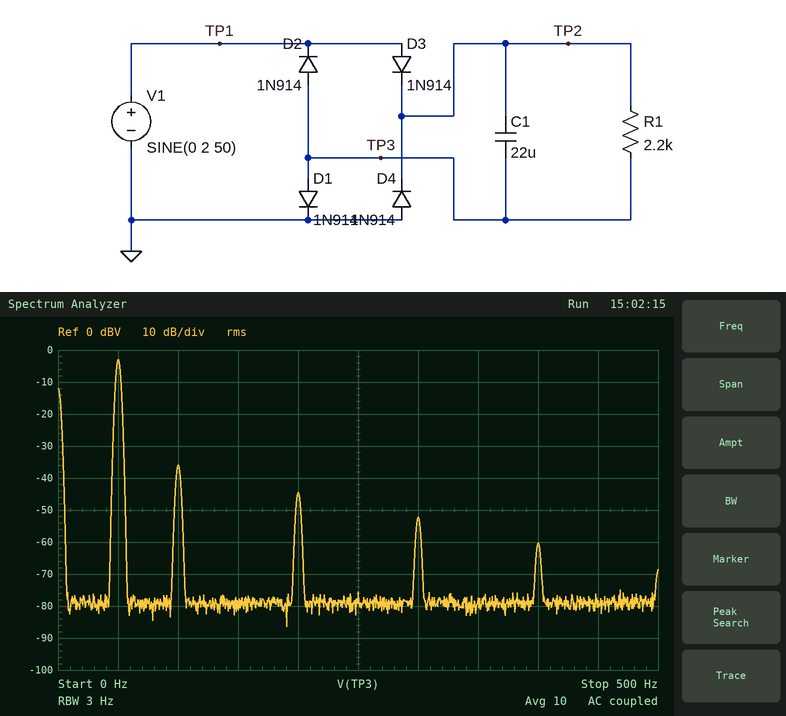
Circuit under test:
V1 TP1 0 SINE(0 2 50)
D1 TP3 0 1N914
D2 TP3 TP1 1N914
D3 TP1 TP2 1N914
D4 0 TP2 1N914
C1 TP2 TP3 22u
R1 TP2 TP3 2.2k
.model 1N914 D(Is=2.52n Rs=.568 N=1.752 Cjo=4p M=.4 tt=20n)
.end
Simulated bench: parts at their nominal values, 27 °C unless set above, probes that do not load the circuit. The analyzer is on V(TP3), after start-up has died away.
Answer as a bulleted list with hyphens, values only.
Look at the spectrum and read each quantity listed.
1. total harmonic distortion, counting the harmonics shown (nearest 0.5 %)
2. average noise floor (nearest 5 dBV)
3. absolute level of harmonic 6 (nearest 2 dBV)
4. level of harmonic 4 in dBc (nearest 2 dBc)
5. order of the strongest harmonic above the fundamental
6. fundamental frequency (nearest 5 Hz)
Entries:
- 2.5 %
- -80 dBV
- -52 dBV
- -42 dBc
- 2
- 50 Hz
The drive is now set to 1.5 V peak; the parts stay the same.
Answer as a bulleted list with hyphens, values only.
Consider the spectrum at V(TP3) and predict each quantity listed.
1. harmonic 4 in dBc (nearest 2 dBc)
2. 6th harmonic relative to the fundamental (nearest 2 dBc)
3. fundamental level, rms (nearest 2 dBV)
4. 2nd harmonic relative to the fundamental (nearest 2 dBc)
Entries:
- -46 dBc
- -56 dBc
- -6 dBV
- -38 dBc
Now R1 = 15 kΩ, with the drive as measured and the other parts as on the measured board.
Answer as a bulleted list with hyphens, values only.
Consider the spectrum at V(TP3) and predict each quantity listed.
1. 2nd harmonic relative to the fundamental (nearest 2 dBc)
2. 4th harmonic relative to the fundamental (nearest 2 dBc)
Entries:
- -48 dBc
- -56 dBc
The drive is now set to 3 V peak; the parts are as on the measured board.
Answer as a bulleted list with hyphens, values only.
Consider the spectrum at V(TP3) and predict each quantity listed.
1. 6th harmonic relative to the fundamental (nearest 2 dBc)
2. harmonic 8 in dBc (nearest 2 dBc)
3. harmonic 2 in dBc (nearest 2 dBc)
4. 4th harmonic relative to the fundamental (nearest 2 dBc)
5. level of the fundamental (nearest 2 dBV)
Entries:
- -44 dBc
- -50 dBc
- -30 dBc
- -38 dBc
- 0 dBV
